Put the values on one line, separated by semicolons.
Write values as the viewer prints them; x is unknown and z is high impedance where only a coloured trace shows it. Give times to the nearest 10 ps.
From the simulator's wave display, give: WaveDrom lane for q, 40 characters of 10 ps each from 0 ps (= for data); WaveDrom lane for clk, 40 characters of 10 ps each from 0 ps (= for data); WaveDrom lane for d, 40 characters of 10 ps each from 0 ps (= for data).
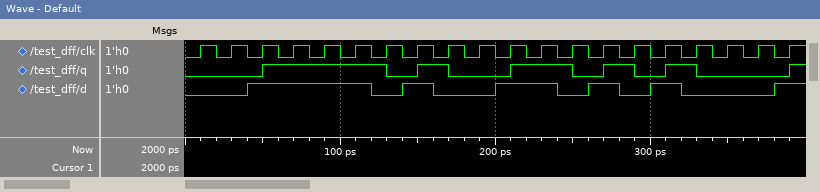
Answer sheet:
{name: 'q', wave: '0....1.......0.1.0...1...0.1.0.1.0.....1'}; {name: 'clk', wave: '0101010101010101010101010101010101010101'}; {name: 'd', wave: '0...1.......0.1.0...1...0.1.0.1.0.....1.'}
